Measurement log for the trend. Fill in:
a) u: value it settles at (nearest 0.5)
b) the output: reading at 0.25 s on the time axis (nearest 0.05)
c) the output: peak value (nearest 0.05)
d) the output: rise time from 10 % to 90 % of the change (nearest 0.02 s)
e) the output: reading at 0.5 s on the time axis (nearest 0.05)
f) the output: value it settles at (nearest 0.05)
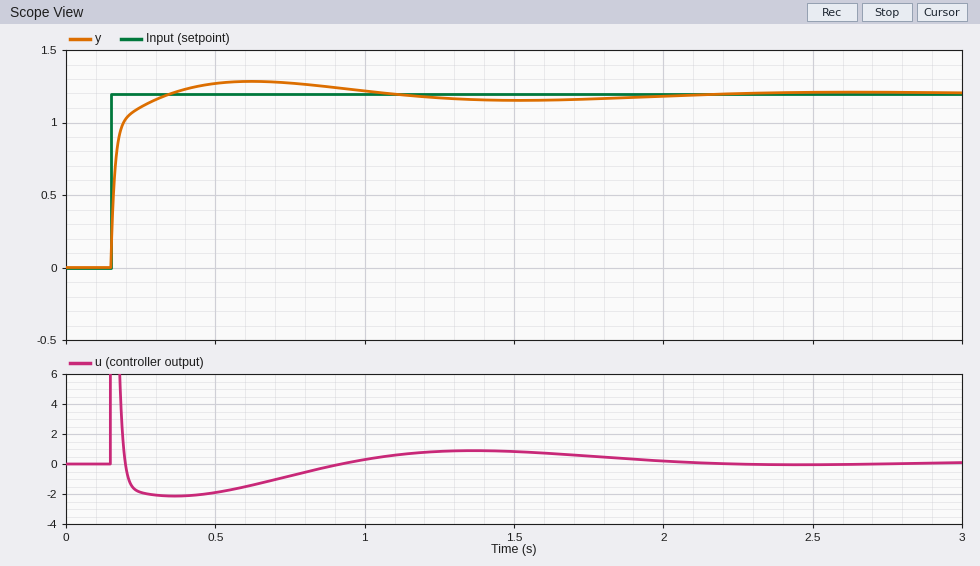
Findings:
0.0
1.10
1.30
0.08 s
1.25
1.20
